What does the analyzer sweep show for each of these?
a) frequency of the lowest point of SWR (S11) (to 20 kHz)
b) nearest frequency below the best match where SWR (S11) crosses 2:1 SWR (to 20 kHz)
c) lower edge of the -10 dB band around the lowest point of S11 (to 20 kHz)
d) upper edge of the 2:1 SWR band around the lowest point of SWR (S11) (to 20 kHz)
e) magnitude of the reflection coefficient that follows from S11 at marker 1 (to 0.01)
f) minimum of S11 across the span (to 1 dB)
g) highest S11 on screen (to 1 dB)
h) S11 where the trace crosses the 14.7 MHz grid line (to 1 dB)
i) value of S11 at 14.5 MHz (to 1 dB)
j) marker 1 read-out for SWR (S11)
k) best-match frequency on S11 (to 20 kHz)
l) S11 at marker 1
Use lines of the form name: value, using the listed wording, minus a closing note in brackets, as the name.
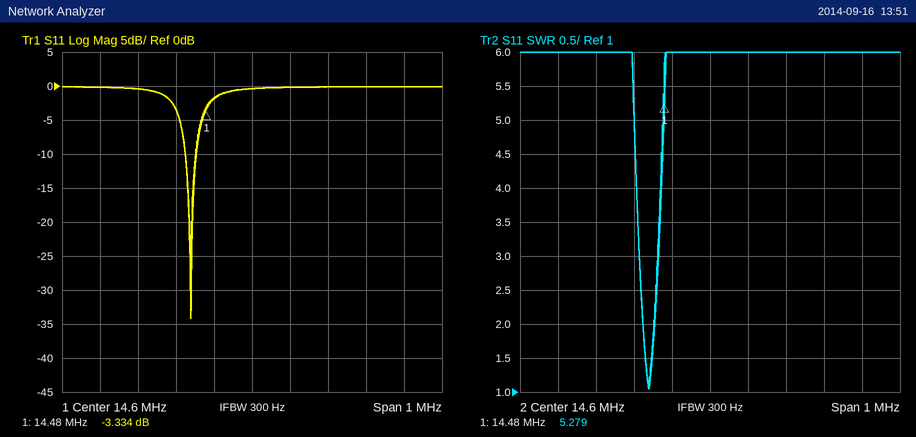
frequency of the lowest point of SWR (S11): 14.44 MHz
nearest frequency below the best match where SWR (S11) crosses 2:1 SWR: 14.42 MHz
lower edge of the -10 dB band around the lowest point of S11: 14.42 MHz
upper edge of the 2:1 SWR band around the lowest point of SWR (S11): 14.46 MHz
magnitude of the reflection coefficient that follows from S11 at marker 1: 0.68
minimum of S11 across the span: -34 dB
highest S11 on screen: 0 dB
S11 where the trace crosses the 14.7 MHz grid line: 0 dB
value of S11 at 14.5 MHz: -2 dB
marker 1 read-out for SWR: 5.279
best-match frequency on S11: 14.44 MHz
S11 at marker 1: -3.334 dB
